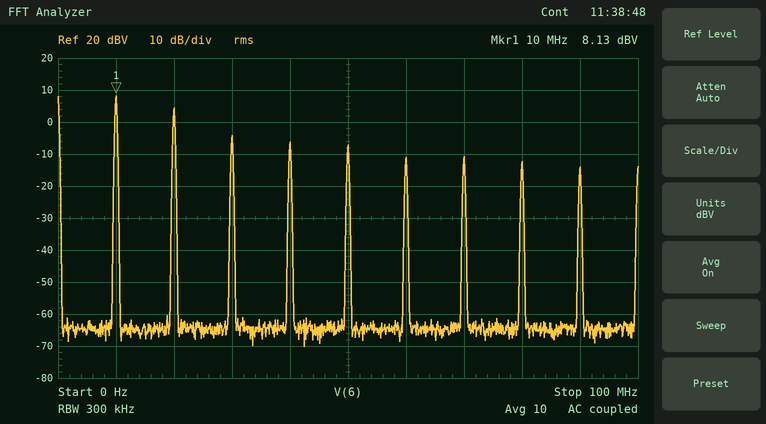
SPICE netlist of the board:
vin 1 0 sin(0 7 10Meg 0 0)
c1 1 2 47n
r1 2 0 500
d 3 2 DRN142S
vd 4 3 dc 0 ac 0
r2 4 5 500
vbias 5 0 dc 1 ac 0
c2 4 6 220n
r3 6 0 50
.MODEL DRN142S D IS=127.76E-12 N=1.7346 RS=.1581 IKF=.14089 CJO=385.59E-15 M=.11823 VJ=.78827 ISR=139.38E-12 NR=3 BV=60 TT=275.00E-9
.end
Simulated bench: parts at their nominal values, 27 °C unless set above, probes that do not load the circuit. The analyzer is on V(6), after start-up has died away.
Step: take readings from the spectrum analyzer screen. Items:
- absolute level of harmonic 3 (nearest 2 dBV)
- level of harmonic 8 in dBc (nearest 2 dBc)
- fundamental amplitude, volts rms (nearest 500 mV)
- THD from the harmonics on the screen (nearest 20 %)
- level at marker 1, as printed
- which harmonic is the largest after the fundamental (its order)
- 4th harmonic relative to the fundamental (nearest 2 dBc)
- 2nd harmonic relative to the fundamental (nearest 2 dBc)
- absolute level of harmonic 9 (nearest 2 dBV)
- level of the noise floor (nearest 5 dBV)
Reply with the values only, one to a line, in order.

-4 dBV
-20 dBc
2.5 V
80 %
8.13 dBV
2
-14 dBc
-4 dBc
-14 dBV
-65 dBV
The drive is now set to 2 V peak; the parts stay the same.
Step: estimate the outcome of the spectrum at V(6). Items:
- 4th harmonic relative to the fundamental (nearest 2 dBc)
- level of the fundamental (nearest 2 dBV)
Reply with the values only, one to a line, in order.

-16 dBc
-2 dBV
